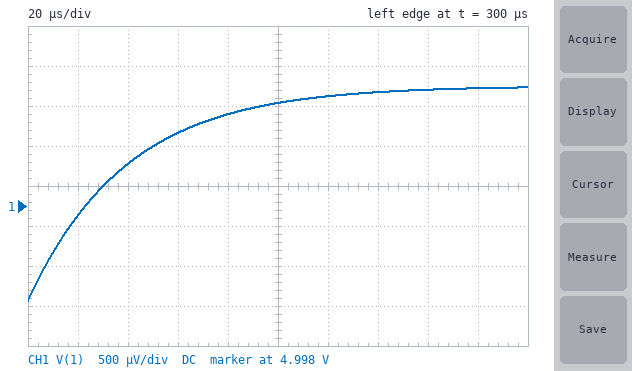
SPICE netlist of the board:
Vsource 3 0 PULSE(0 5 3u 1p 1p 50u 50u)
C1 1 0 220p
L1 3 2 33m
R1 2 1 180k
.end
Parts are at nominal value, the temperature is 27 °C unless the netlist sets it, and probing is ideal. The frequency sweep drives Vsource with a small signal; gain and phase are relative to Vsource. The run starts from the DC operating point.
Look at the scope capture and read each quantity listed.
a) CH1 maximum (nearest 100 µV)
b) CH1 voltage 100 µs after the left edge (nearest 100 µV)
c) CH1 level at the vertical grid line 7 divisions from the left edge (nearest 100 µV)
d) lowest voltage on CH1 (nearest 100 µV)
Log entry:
5.0000 V
4.9998 V
4.9999 V
4.9973 V
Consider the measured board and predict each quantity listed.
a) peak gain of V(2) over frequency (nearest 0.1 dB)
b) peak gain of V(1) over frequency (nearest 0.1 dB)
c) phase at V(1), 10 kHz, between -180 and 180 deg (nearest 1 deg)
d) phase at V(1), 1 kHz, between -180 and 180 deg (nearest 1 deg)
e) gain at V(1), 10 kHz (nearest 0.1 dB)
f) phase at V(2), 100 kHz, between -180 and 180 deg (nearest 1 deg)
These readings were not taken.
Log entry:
0 dB
0 dB
-69 deg
-14 deg
-8.5 dB
-7 deg
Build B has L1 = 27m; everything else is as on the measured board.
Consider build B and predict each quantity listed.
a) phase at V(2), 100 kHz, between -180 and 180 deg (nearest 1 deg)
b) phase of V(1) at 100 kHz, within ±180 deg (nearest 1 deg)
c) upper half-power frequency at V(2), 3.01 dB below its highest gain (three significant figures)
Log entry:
-5 deg
-93 deg
1.06 MHz
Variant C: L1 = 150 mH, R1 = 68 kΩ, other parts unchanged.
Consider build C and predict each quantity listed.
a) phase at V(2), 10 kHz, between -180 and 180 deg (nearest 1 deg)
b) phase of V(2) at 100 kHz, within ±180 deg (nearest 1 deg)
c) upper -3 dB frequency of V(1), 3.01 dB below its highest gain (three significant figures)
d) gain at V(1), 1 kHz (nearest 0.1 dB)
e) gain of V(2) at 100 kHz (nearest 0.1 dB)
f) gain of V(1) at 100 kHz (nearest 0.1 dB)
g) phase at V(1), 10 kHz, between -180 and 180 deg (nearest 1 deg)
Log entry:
-4 deg
-58 deg
12.4 kHz
0 dB
-4.2 dB
-23.7 dB
-47 deg
